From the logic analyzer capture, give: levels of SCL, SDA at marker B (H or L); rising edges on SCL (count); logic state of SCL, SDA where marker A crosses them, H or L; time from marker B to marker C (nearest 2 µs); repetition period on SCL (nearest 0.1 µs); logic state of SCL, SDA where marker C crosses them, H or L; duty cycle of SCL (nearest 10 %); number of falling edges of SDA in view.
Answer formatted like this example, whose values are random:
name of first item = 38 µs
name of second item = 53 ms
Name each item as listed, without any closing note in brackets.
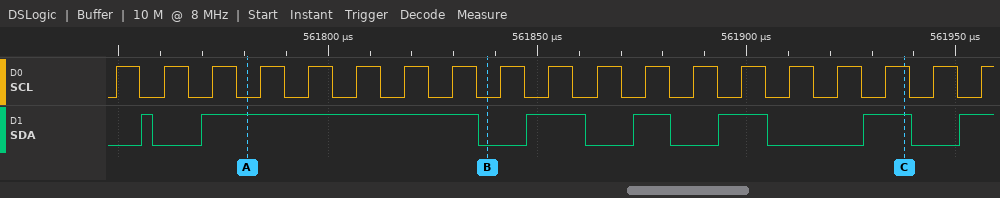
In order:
levels of SCL, SDA at marker B = SCL=L, SDA=L
rising edges on SCL = 19
logic state of SCL, SDA where marker A crosses them, H or L = SCL=L, SDA=H
time from marker B to marker C = 100 µs
repetition period on SCL = 11.5 µs
logic state of SCL, SDA where marker C crosses them, H or L = SCL=H, SDA=H
duty cycle of SCL = 50 %
number of falling edges of SDA in view = 6
